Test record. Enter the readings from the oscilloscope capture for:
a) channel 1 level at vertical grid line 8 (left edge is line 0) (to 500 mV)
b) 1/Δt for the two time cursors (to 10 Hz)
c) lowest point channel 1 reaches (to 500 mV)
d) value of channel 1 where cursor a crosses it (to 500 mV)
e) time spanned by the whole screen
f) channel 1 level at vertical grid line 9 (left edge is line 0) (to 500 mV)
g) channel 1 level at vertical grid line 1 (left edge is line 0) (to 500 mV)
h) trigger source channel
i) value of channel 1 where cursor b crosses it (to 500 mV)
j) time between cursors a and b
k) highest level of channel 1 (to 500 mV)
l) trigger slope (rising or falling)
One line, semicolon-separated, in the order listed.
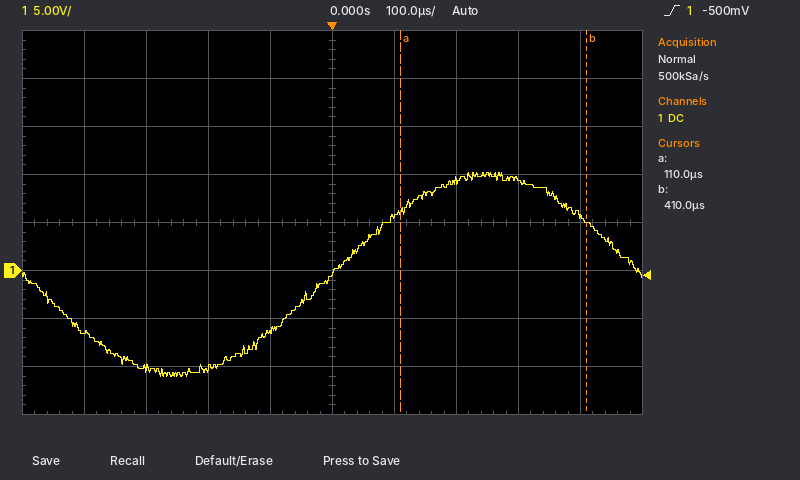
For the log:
9.5 V; 3.33 kHz; -11.0 V; 6.0 V; 1 ms; 6.0 V; -6.5 V; channel 1; 5.0 V; 300 µs; 10.0 V; rising
